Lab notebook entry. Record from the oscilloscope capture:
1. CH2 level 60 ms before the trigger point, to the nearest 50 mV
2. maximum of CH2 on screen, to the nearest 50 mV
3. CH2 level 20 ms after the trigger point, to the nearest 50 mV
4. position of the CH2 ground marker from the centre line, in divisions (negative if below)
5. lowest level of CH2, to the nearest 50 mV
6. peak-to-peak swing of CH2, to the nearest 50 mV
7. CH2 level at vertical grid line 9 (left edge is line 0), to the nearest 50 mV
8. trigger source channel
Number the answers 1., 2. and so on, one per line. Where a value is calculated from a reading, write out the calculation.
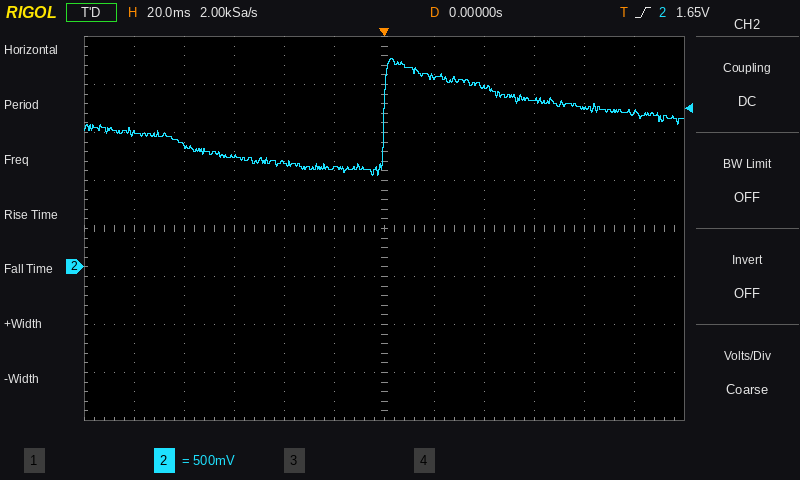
1. 1.15 V
2. 2.15 V
3. 2.00 V
4. -0.8 div
5. 950 mV
6. 2.15 V − (950 mV) = 1.20 V
7. 1.75 V
8. CH2
